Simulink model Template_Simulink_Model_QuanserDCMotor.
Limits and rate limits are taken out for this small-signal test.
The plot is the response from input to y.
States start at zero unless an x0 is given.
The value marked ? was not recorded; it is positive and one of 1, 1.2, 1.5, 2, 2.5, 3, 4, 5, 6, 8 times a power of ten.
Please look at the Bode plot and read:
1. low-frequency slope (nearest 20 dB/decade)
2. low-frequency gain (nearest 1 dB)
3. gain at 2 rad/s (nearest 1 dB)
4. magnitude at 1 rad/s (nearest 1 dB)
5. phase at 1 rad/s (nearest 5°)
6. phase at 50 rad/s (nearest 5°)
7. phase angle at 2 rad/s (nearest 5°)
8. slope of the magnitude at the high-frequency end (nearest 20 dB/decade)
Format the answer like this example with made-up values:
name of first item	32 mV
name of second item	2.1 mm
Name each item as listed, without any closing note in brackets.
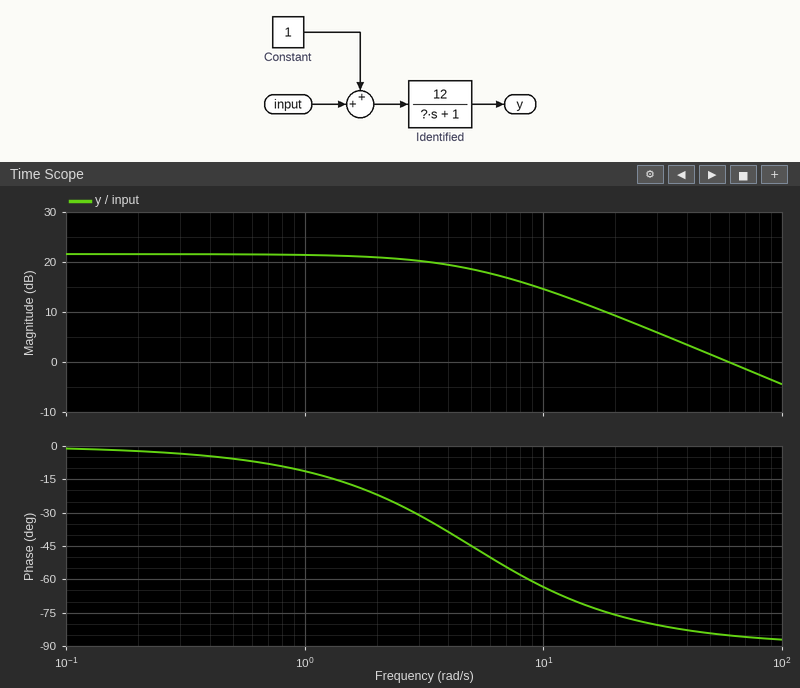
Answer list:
low-frequency slope	0 dB/decade
low-frequency gain	22 dB
gain at 2 rad/s	21 dB
magnitude at 1 rad/s	21 dB
phase at 1 rad/s	-10°
phase at 50 rad/s	-85°
phase angle at 2 rad/s	-20°
slope of the magnitude at the high-frequency end	-20 dB/decade
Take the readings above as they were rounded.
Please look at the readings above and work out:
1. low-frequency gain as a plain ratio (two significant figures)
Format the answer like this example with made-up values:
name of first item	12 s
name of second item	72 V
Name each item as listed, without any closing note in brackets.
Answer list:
low-frequency gain as a plain ratio	13
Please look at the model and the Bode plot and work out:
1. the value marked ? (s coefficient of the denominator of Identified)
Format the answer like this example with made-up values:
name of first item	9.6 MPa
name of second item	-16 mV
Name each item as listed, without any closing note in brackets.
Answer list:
the value marked ?	0.2
